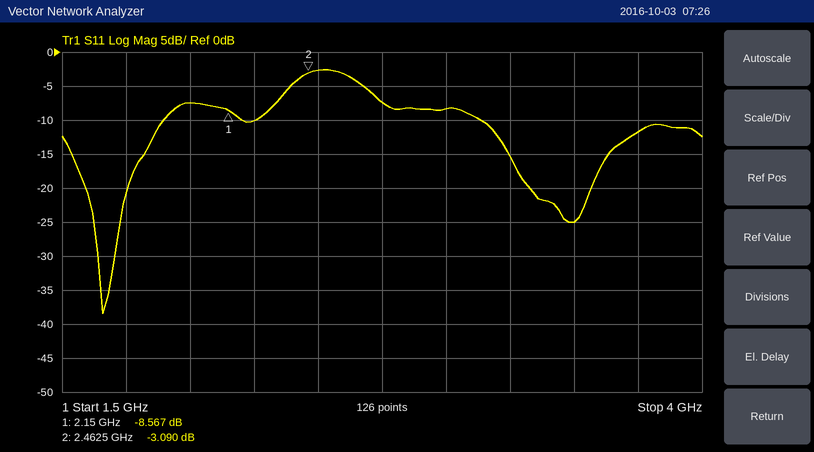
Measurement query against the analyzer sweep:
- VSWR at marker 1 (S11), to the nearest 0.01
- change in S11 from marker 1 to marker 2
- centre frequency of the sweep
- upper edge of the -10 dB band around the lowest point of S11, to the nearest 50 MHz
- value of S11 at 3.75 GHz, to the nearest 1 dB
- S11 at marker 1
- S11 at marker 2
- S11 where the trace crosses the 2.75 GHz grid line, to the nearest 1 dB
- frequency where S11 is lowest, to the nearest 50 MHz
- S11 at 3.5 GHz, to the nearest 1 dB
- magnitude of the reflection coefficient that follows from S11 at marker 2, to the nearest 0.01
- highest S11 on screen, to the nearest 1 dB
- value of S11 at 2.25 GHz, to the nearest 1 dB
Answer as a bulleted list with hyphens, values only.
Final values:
- 2.19
- 5.477 dB
- 2.75 GHz
- 1.90 GHz
- -12 dB
- -8.567 dB
- -3.090 dB
- -7 dB
- 1.65 GHz
- -25 dB
- 0.70
- -3 dB
- -10 dB
